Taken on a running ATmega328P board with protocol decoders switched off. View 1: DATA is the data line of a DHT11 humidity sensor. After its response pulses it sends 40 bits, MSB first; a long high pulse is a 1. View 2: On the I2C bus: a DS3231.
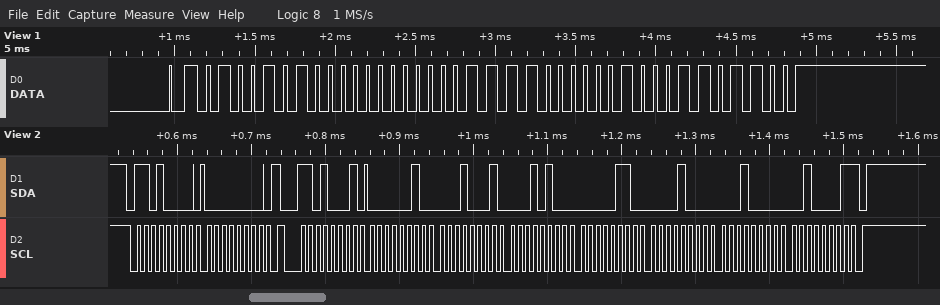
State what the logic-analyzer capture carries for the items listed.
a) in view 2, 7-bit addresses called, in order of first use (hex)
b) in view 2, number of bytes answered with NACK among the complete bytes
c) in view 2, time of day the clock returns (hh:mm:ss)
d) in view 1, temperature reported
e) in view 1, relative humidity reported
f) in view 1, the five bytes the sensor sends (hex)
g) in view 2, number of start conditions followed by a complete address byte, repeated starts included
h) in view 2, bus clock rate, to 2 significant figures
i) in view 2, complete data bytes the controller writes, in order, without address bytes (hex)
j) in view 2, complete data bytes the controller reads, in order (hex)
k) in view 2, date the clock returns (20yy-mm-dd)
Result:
0x68
1
14:11:02
30.4 °C
74 %
4A 00 1E 04 6C
2
100 kHz
00
02 11 14 06 08 10 21
2021-10-08
